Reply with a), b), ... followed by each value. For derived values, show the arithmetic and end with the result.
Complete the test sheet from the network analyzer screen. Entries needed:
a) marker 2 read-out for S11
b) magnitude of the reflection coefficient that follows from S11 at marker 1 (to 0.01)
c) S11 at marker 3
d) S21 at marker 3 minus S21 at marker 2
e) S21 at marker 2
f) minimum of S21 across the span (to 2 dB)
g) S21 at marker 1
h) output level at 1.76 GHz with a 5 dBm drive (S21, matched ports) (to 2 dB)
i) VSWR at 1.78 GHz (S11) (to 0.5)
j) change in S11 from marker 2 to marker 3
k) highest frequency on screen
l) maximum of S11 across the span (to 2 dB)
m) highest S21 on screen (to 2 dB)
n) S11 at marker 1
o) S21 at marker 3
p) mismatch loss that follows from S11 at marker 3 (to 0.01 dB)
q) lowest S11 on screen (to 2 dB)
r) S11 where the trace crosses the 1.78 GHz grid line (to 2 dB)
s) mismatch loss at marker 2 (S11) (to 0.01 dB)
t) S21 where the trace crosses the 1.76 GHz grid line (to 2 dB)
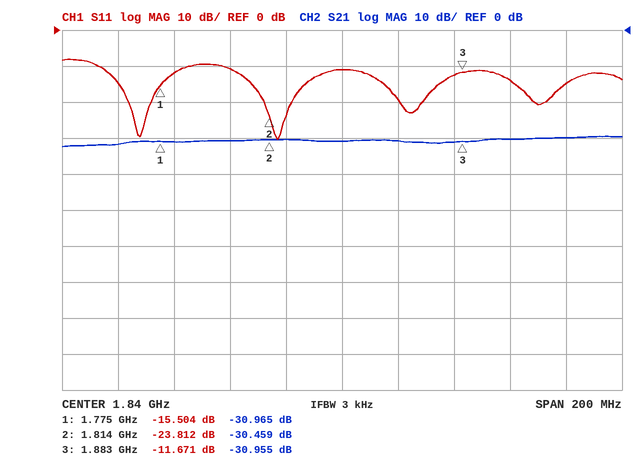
a) -23.812 dB
b) 10^(-15.504/20) ≈ 0.17
c) -11.671 dB
d) -30.955 − (-30.459) = -0.496 dB
e) -30.459 dB
f) -32 dB
g) -30.965 dB
h) 5 dBm + (-32 dB) = -26 dBm
i) |Γ| = 10^(-12/20) = 0.2512; VSWR = (1 + 0.2512)/(1 − 0.2512) ≈ 1.67, so 1.5 to the nearest 0.5
j) -11.671 − (-23.812) = 12.141 dB
k) 1.94 GHz
l) -8 dB
m) -30 dB
n) -15.504 dB
o) -30.955 dB
p) −10 log10(1 − 10^(-11.671/10)) ≈ 0.31 dB
q) -30 dB
r) -12 dB
s) −10 log10(1 − 10^(-23.812/10)) ≈ 0.02 dB
t) -32 dB
